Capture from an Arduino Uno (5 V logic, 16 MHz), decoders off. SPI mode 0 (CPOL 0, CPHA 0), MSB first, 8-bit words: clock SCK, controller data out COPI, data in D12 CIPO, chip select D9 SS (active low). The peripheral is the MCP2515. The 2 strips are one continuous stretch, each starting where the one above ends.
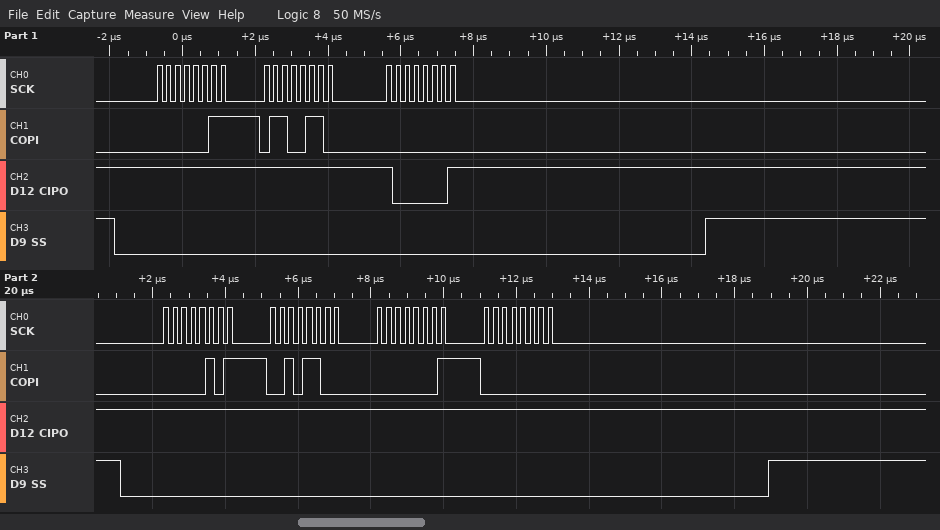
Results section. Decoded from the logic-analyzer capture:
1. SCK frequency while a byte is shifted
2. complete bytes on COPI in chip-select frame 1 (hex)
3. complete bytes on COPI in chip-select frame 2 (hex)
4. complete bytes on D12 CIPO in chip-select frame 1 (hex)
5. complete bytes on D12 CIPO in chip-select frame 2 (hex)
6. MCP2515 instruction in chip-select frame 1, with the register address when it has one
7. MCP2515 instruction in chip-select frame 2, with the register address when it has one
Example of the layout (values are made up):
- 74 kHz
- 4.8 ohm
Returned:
- 4 MHz
- 03 66 00
- 05 2C 01 00
- FF FF 81
- FF FF FF FF
- READ 0x66
- BIT MODIFY 0x2C
